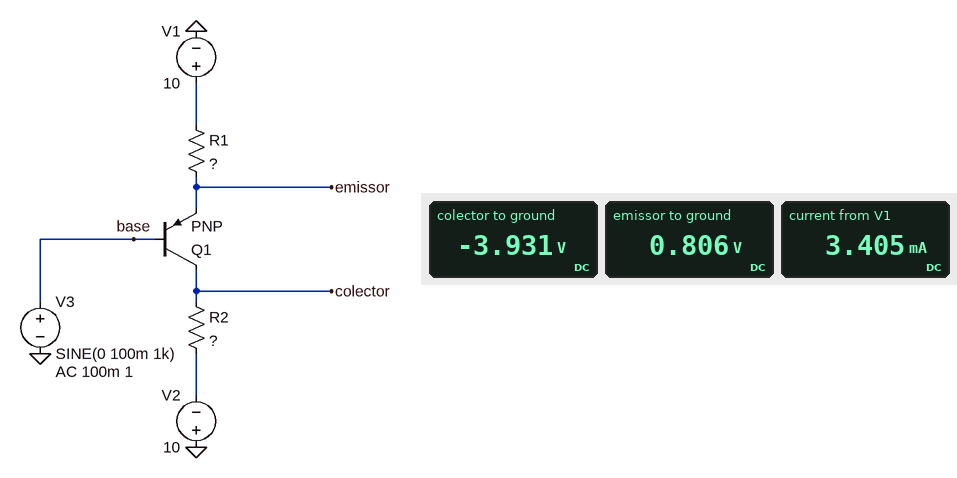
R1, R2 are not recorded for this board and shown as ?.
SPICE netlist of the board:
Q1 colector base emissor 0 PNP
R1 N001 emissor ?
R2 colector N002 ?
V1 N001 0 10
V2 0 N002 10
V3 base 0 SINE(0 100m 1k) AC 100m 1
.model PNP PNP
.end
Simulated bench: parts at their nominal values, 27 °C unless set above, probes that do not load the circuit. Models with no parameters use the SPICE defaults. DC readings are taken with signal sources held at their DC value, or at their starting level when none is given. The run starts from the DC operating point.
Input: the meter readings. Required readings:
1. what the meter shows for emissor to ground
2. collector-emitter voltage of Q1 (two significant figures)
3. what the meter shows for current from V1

0.806 V
-4.7 V
3.405 mA
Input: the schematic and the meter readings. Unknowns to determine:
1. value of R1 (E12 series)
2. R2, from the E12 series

2.7 kΩ
1.8 kΩ
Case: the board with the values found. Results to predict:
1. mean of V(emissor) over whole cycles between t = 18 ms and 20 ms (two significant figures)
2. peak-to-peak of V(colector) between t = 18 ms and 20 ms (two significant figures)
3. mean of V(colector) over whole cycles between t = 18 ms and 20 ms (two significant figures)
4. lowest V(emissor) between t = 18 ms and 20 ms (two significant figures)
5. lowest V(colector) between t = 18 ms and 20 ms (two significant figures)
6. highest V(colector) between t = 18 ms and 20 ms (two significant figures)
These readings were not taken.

810 mV
130 mV
-3.9 V
710 mV
-4.0 V
-3.9 V
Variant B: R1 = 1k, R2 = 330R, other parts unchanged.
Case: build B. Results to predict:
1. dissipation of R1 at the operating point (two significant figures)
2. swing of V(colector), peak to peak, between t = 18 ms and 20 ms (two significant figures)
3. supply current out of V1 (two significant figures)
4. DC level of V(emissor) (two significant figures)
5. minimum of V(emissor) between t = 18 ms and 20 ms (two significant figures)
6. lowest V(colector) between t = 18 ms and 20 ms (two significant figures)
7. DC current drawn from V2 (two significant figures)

84 mW
65 mV
9.2 mA
830 mV
730 mV
-7.0 V
9.1 mA
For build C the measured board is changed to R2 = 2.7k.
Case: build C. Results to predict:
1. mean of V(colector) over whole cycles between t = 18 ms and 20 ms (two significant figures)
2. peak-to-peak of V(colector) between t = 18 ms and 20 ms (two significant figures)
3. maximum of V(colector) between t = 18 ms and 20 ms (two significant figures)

-900 mV
200 mV
-800 mV
